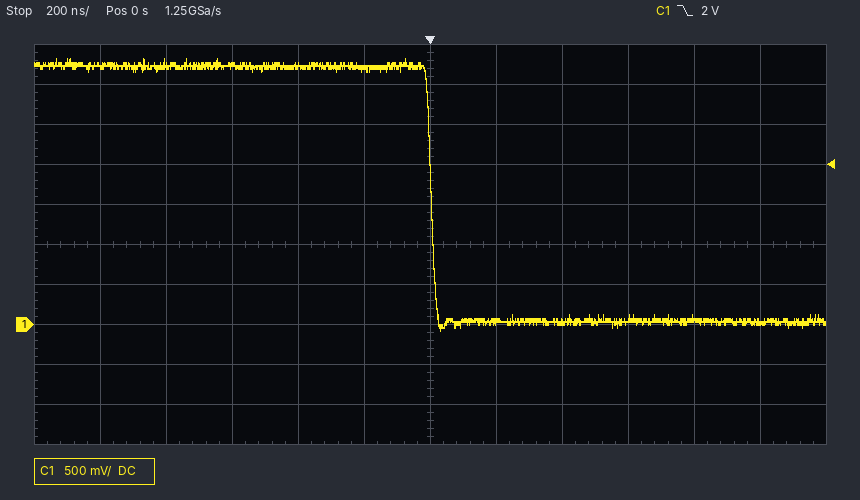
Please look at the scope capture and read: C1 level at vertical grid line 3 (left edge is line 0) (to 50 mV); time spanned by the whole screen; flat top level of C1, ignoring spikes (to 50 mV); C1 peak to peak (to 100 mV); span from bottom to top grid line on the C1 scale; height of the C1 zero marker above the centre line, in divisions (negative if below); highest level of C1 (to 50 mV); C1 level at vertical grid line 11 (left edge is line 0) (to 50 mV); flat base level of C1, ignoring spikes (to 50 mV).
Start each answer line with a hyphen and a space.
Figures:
- 3.25 V
- 2.4 µs
- 3.25 V
- 3.40 V
- 5 V
- -2.0 div
- 3.30 V
- 50 mV
- 50 mV
